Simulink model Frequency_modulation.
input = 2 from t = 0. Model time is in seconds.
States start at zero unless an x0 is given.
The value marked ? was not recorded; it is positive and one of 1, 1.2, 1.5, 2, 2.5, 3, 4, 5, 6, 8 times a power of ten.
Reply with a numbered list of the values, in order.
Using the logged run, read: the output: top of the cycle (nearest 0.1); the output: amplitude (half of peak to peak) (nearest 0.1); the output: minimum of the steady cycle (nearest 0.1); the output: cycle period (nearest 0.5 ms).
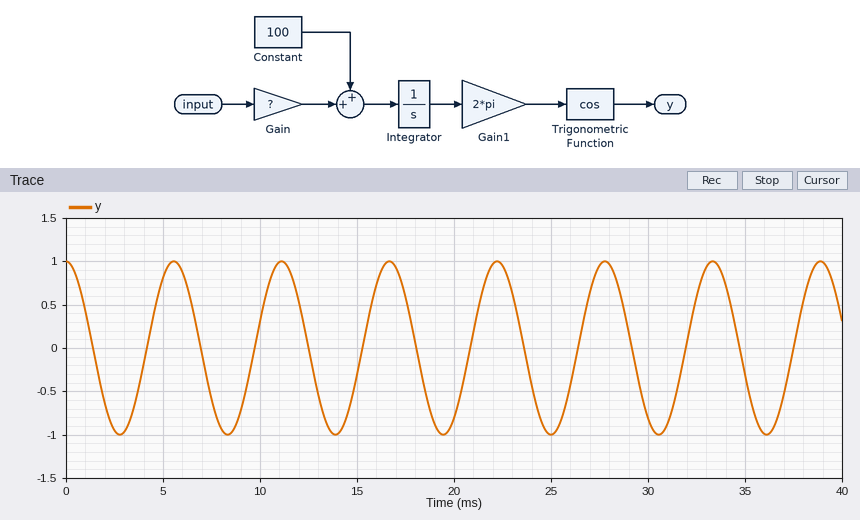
1. 1.0
2. 1.0
3. -1.0
4. 5.5 ms
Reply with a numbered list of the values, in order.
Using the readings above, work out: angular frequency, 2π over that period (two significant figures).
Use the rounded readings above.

1. 1.1 rad/ms
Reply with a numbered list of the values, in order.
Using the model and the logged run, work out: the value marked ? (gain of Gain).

1. 40
